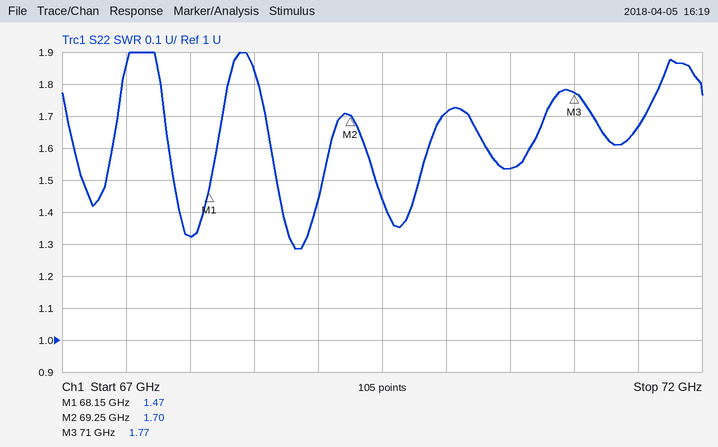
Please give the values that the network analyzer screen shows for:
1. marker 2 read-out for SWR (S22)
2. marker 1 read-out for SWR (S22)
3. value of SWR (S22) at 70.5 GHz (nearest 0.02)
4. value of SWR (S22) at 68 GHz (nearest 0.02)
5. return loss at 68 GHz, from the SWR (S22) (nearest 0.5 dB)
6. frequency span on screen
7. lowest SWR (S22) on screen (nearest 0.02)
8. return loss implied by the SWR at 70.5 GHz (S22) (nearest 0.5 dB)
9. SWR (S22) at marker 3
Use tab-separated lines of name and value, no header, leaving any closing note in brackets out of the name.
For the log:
marker 2 read-out for SWR	1.70
marker 1 read-out for SWR	1.47
value of SWR (S22) at 70.5 GHz	1.54
value of SWR (S22) at 68 GHz	1.32
return loss at 68 GHz, from the SWR (S22)	17.0 dB
frequency span on screen	5 GHz
lowest SWR (S22) on screen	1.28
return loss implied by the SWR at 70.5 GHz (S22)	13.5 dB
SWR (S22) at marker 3	1.77
